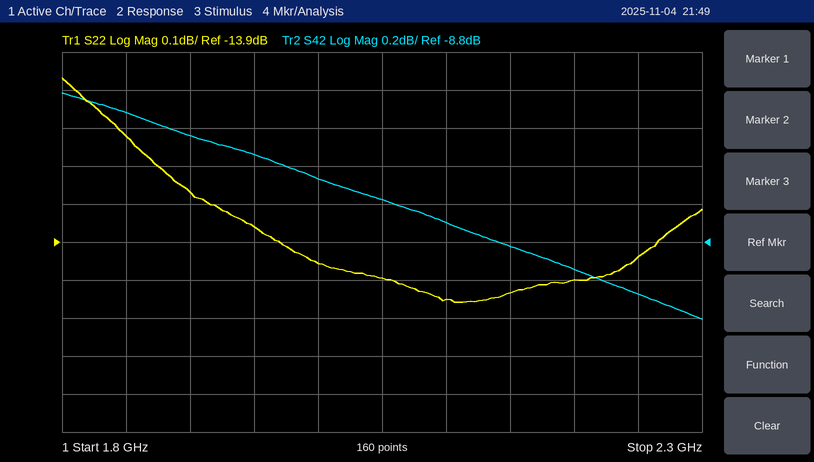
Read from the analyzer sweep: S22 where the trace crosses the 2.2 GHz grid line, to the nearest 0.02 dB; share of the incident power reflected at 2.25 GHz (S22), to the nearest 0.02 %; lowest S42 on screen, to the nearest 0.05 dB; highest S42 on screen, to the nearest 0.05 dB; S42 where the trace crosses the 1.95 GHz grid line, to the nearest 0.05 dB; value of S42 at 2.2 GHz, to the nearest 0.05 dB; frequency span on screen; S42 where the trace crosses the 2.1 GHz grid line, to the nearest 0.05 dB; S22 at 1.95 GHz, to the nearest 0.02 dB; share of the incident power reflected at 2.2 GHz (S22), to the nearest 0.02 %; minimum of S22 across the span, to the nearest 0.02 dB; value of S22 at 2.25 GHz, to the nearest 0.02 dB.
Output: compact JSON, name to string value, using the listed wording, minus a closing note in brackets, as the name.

{"S22 where the trace crosses the 2.2 GHz grid line, to the nearest 0.02 dB": "-14.00 dB", "share of the incident power reflected at 2.25 GHz (S22), to the nearest 0.02 %": "4.04 %", "lowest S42 on screen, to the nearest 0.05 dB": "-9.20 dB", "highest S42 on screen, to the nearest 0.05 dB": "-8.00 dB", "S42 where the trace crosses the 1.95 GHz grid line, to the nearest 0.05 dB": "-8.35 dB", "value of S42 at 2.2 GHz, to the nearest 0.05 dB": "-8.95 dB", "frequency span on screen": "500 MHz", "S42 where the trace crosses the 2.1 GHz grid line, to the nearest 0.05 dB": "-8.70 dB", "S22 at 1.95 GHz, to the nearest 0.02 dB": "-13.86 dB", "share of the incident power reflected at 2.2 GHz (S22), to the nearest 0.02 %": "3.98 %", "minimum of S22 across the span, to the nearest 0.02 dB": "-14.06 dB", "value of S22 at 2.25 GHz, to the nearest 0.02 dB": "-13.94 dB"}
